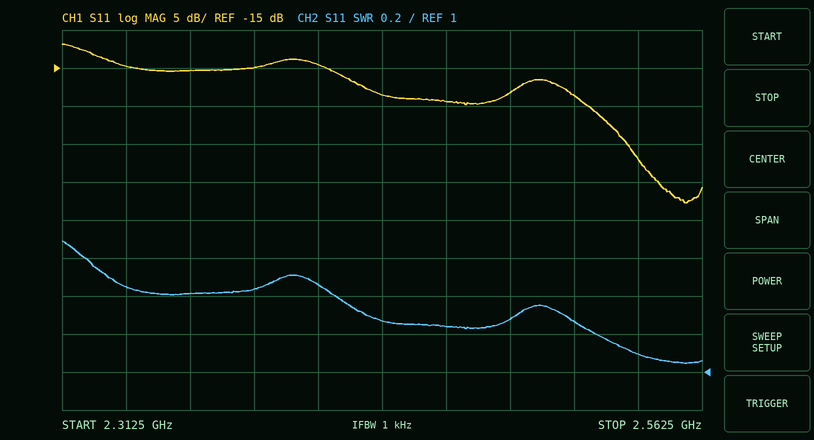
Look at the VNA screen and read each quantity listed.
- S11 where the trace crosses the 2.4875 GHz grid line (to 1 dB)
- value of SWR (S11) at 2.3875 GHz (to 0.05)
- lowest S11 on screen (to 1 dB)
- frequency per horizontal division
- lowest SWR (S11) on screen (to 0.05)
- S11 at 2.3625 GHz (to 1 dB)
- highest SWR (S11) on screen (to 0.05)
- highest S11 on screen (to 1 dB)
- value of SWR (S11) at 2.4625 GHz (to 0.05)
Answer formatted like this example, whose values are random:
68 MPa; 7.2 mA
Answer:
-18 dB; 1.45; -33 dB; 25 MHz; 1.05; -15 dB; 1.70; -12 dB; 1.25
